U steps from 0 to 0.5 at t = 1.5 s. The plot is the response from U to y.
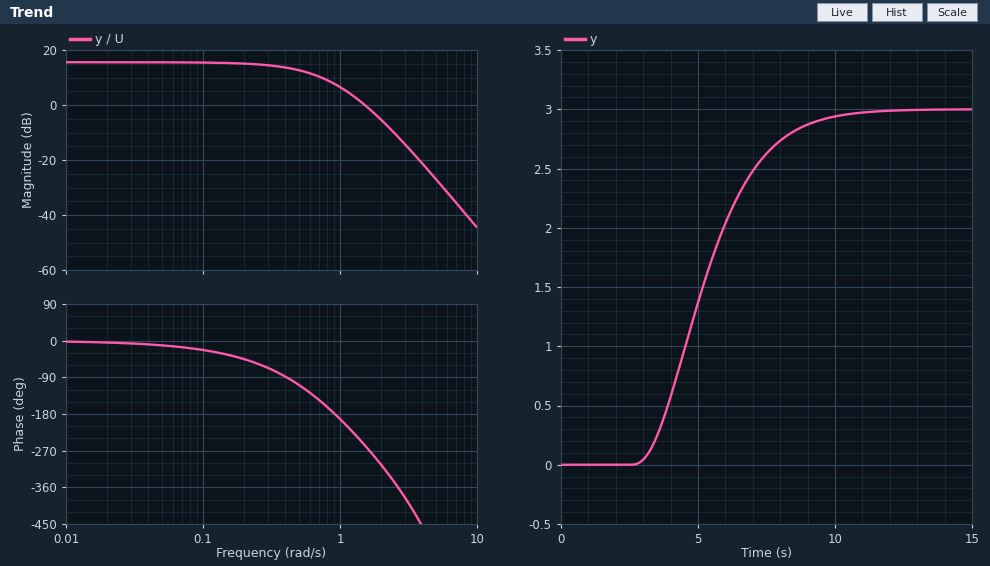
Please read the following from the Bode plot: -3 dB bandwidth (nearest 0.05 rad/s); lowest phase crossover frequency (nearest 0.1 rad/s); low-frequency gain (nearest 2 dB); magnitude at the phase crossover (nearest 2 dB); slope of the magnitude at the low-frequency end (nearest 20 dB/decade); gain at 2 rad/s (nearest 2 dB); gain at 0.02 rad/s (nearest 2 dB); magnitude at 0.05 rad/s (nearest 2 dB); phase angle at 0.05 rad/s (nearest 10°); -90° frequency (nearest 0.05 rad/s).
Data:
0.50 rad/s
0.9 rad/s
16 dB
8 dB
0 dB/decade
-6 dB
16 dB
16 dB
-10°
0.40 rad/s
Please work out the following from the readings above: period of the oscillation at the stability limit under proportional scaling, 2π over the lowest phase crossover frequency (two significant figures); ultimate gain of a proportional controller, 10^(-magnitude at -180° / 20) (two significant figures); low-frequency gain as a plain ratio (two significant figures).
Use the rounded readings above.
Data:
7.0 s
0.40
6.3
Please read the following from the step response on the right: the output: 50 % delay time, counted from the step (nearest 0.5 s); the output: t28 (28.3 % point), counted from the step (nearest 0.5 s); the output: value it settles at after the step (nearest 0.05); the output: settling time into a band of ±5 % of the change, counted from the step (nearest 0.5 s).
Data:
3.5 s
3.0 s
3.00
7.5 s
